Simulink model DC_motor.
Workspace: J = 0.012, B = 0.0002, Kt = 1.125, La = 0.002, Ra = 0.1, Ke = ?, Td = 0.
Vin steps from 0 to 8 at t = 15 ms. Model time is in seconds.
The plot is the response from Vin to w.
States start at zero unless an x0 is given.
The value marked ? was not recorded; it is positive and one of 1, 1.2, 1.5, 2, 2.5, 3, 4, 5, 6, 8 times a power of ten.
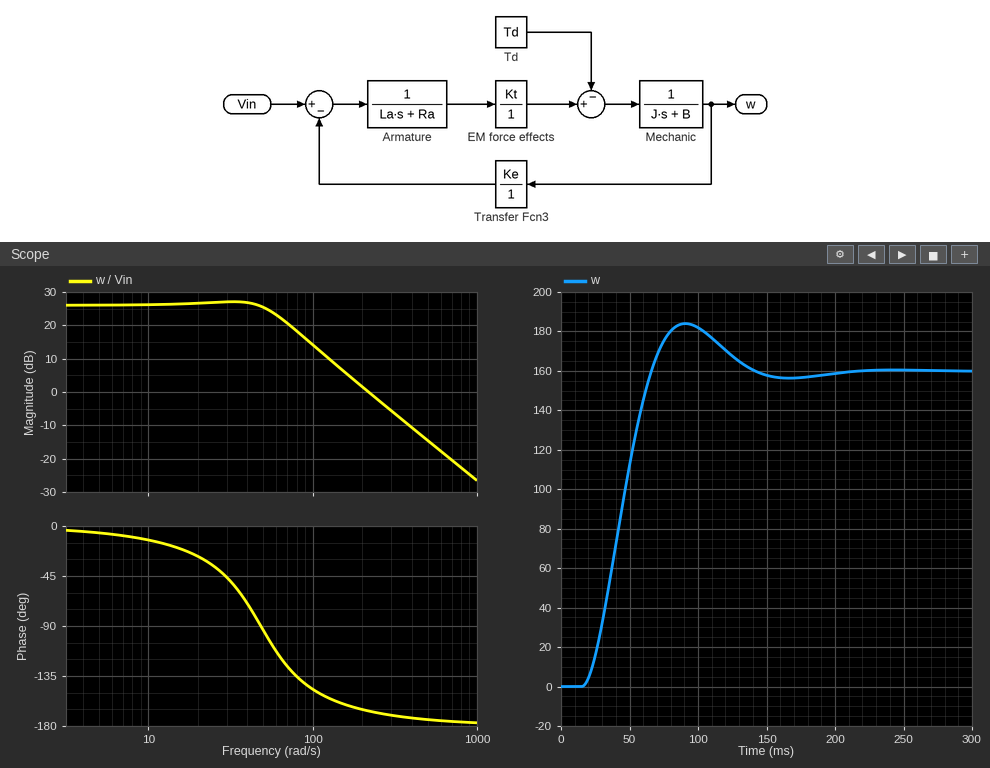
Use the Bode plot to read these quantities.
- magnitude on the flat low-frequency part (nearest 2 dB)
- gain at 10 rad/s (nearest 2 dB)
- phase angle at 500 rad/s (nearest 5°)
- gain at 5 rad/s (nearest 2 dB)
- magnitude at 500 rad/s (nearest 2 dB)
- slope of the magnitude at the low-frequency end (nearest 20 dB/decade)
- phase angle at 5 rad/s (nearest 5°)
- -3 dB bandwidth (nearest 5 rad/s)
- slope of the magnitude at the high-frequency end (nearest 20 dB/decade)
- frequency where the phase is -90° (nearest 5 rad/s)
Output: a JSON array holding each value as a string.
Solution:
["26 dB", "26 dB", "-175°", "26 dB", "-14 dB", "0 dB/decade", "-5°", "60 rad/s", "-40 dB/decade", "50 rad/s"]
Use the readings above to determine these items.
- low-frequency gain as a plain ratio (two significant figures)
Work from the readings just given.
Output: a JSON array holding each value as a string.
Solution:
["20"]
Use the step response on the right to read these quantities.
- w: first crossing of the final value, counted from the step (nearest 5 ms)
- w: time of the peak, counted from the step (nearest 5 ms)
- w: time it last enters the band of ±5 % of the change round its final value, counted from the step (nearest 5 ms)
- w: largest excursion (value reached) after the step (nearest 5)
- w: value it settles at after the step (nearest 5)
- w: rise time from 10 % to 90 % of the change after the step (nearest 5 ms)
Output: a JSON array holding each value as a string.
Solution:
["50 ms", "75 ms", "110 ms", "185", "160", "35 ms"]
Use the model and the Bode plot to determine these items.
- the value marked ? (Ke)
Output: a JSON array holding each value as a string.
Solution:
["0.05"]
